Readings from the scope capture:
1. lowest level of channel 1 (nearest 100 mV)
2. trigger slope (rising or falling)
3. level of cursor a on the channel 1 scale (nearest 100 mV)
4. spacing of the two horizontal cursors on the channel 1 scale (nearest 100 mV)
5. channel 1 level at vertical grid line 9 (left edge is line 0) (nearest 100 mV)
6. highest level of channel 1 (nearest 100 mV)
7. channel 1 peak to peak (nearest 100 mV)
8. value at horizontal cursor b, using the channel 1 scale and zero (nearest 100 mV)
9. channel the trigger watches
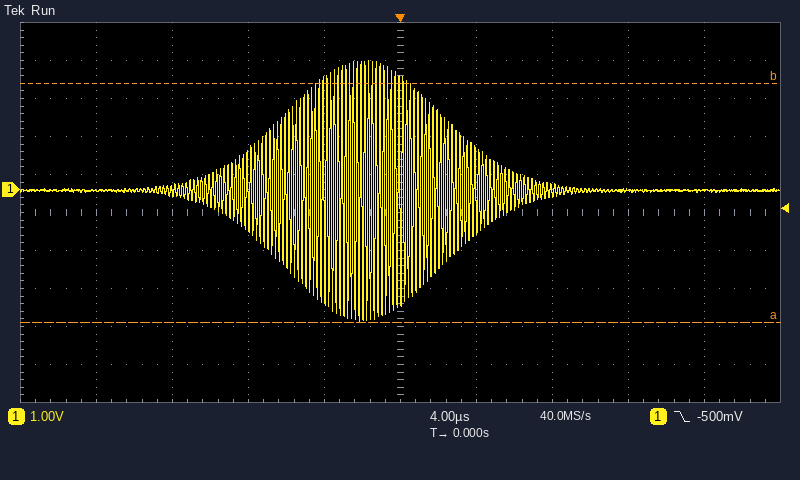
-3.5 V
falling
-3.5 V
6.3 V
0.0 V
3.4 V
6.9 V
2.8 V
channel 1
